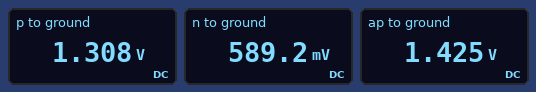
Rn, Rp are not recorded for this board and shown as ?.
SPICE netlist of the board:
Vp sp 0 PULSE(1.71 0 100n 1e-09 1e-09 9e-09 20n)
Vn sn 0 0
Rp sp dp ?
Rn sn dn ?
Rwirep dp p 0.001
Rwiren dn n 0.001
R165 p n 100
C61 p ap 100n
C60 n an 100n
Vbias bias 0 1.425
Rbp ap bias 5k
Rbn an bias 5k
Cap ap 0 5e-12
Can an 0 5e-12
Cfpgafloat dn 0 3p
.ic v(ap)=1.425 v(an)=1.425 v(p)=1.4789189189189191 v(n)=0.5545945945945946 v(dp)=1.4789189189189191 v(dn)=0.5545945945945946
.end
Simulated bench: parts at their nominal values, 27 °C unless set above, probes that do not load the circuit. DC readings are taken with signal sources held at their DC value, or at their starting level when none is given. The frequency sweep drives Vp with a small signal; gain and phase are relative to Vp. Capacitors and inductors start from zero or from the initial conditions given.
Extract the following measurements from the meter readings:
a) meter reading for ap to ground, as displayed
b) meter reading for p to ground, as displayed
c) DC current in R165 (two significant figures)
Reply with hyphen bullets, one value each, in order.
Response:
- 1.425 V
- 1.308 V
- 7.2 mA
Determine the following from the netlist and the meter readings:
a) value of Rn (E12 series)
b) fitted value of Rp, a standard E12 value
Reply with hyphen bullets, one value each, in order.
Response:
- 82 Ω
- 56 Ω
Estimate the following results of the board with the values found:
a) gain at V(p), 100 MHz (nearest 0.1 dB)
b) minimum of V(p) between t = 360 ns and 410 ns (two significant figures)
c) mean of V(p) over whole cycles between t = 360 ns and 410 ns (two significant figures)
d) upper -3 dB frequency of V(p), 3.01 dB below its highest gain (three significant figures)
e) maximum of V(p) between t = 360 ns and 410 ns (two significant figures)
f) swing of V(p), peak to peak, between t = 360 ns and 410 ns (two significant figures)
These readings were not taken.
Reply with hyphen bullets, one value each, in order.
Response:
- -2.6 dB
- 15 mV
- 660 mV
- 581 MHz
- 1.3 V
- 1.3 V
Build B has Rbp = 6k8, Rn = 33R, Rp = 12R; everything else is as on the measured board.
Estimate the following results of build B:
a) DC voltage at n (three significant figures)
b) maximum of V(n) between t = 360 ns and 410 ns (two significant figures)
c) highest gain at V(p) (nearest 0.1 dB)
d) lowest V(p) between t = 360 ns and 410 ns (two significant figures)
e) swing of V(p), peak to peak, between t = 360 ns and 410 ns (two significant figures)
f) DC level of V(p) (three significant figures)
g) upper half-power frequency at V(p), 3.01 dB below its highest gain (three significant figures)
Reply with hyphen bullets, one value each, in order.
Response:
- 389 mV
- 390 mV
- -0.8 dB
- 2.7 mV
- 1.6 V
- 1.57 V
- 2.80 GHz
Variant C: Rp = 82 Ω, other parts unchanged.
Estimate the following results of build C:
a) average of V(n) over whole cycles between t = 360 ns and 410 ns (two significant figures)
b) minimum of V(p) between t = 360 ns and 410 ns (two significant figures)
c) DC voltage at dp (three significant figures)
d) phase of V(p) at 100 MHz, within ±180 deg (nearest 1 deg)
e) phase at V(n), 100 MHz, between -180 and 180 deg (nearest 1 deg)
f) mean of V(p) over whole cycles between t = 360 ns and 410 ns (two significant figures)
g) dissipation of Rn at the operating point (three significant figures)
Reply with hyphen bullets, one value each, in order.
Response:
- 270 mV
- 19 mV
- 1.18 V
- -13 deg
- -25 deg
- 600 mV
- 3.44 mW
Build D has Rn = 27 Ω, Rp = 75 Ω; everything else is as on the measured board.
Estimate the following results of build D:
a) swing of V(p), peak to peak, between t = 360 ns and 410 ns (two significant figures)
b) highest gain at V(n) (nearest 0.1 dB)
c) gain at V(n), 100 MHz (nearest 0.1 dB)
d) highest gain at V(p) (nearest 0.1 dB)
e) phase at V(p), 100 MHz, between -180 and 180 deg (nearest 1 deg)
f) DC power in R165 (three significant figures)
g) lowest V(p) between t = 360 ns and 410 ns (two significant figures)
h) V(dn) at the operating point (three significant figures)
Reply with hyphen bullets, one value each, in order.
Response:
- 1.1 V
- -17.6 dB
- -17.8 dB
- -4.1 dB
- -9 deg
- 7.17 mW
- 15 mV
- 229 mV
